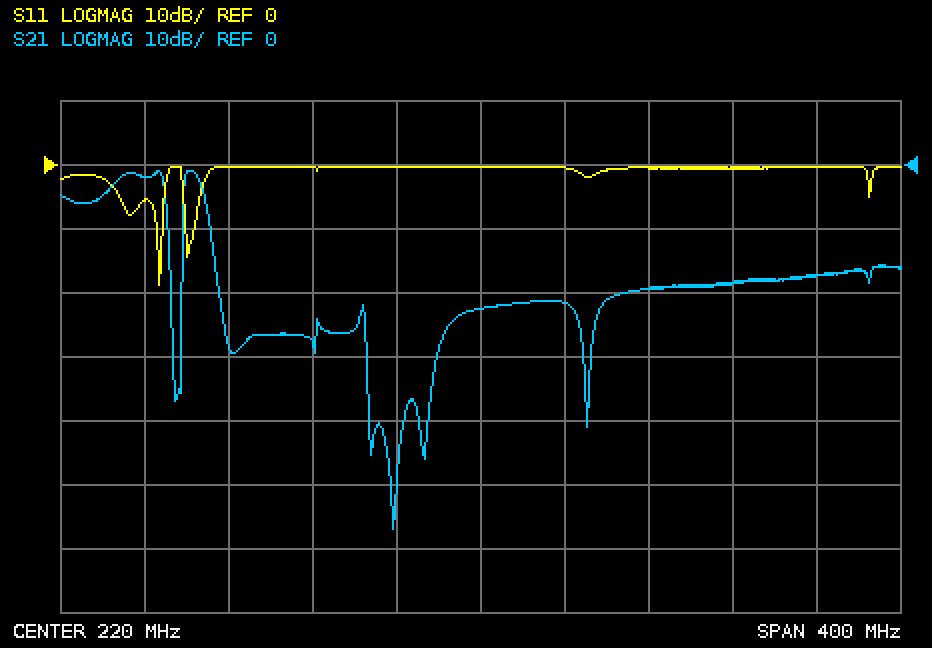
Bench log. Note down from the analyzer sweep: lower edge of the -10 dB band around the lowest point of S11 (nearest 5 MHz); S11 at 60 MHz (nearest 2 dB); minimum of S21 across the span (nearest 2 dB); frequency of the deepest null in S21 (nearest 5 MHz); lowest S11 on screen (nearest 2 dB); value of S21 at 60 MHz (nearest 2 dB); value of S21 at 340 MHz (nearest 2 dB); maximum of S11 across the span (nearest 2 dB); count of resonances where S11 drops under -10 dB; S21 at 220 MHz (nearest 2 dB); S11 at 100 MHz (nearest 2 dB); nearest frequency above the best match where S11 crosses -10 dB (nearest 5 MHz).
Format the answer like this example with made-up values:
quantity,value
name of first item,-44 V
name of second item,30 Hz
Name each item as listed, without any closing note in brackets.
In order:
quantity,value
lower edge of the -10 dB band around the lowest point of S11,65 MHz
S11 at 60 MHz,-6 dB
minimum of S21 across the span,-56 dB
frequency of the deepest null in S21,180 MHz
lowest S11 on screen,-18 dB
value of S21 at 60 MHz,-2 dB
value of S21 at 340 MHz,-18 dB
maximum of S11 across the span,0 dB
count of resonances where S11 drops under -10 dB,2
S21 at 220 MHz,-22 dB
S11 at 100 MHz,0 dB
nearest frequency above the best match where S11 crosses -10 dB,70 MHz
